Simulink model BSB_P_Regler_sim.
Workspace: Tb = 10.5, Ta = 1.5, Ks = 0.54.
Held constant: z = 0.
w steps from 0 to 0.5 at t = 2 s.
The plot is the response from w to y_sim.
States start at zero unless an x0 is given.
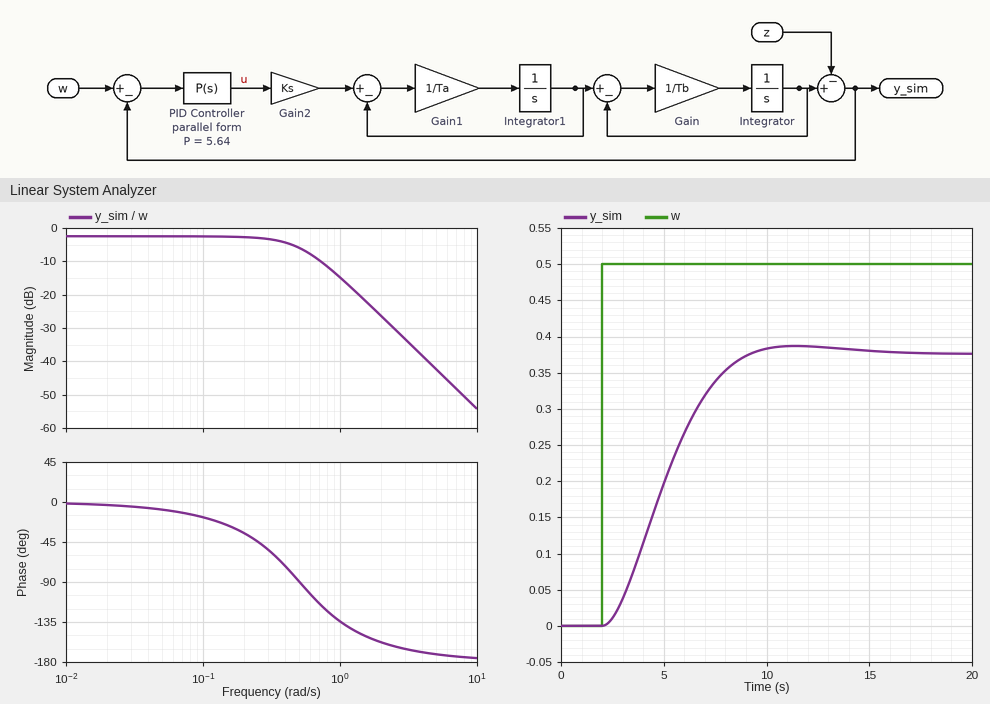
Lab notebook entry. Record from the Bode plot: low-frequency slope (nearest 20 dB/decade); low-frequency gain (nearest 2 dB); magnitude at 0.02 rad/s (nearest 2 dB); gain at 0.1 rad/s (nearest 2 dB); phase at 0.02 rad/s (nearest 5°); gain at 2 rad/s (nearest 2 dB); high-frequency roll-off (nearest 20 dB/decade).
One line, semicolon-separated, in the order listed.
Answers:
0 dB/decade; -2 dB; -2 dB; -2 dB; -5°; -26 dB; -40 dB/decade
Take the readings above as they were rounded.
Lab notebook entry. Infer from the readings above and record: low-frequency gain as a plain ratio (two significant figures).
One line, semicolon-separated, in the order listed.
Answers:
0.79
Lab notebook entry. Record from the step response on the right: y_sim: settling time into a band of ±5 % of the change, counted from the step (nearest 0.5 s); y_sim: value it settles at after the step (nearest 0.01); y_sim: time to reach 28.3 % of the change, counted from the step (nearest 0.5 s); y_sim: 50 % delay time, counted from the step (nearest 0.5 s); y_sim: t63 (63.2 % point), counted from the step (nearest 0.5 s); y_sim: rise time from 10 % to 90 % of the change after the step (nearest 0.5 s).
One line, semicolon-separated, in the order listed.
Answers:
6.0 s; 0.38; 2.0 s; 3.0 s; 3.5 s; 4.5 s
